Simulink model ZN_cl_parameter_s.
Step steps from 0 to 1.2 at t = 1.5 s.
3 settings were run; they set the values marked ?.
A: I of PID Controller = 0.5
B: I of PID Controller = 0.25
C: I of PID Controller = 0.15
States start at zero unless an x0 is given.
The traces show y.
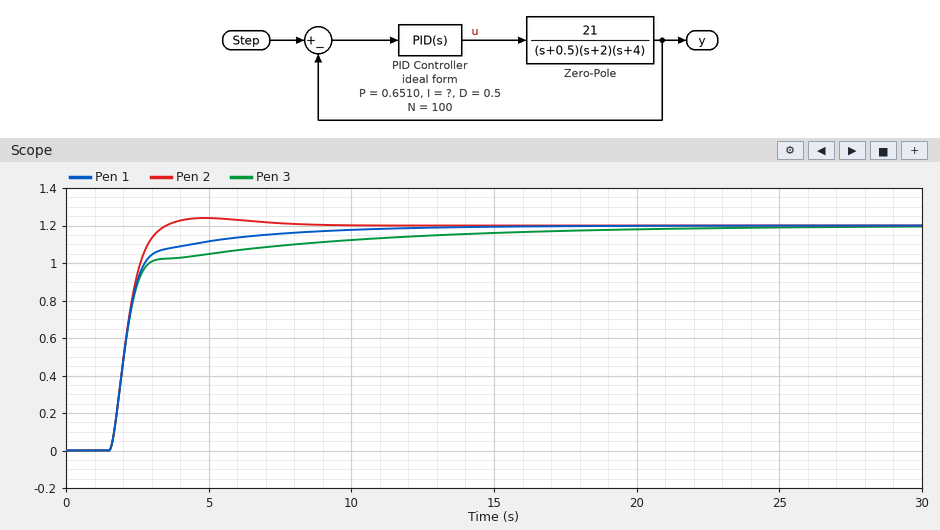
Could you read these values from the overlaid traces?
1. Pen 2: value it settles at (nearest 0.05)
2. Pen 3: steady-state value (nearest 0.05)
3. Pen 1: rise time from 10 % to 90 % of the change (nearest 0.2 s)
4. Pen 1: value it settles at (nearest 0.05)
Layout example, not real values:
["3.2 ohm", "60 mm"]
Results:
["1.20", "1.20", "2.0 s", "1.20"]
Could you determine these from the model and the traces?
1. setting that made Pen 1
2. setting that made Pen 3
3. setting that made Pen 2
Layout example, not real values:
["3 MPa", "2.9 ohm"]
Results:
["B", "C", "A"]
